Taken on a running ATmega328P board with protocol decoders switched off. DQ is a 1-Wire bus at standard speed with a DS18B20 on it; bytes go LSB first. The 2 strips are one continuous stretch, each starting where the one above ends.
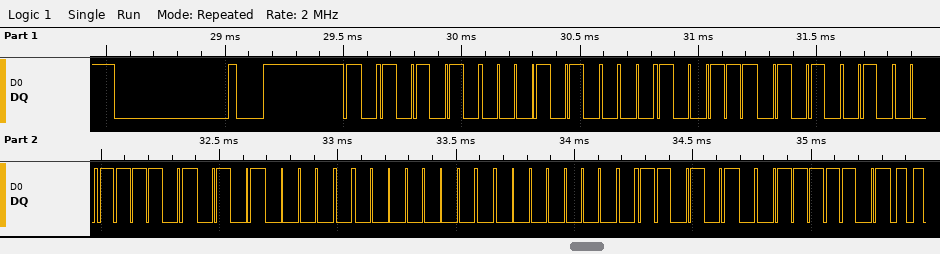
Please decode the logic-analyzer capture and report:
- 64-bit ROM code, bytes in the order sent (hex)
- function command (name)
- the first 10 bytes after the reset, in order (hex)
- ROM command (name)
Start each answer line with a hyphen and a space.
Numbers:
- 28 E4 4A BC 0A 00 00 56
- Read Scratchpad
- 55 28 E4 4A BC 0A 00 00 56 BE
- Match ROM
